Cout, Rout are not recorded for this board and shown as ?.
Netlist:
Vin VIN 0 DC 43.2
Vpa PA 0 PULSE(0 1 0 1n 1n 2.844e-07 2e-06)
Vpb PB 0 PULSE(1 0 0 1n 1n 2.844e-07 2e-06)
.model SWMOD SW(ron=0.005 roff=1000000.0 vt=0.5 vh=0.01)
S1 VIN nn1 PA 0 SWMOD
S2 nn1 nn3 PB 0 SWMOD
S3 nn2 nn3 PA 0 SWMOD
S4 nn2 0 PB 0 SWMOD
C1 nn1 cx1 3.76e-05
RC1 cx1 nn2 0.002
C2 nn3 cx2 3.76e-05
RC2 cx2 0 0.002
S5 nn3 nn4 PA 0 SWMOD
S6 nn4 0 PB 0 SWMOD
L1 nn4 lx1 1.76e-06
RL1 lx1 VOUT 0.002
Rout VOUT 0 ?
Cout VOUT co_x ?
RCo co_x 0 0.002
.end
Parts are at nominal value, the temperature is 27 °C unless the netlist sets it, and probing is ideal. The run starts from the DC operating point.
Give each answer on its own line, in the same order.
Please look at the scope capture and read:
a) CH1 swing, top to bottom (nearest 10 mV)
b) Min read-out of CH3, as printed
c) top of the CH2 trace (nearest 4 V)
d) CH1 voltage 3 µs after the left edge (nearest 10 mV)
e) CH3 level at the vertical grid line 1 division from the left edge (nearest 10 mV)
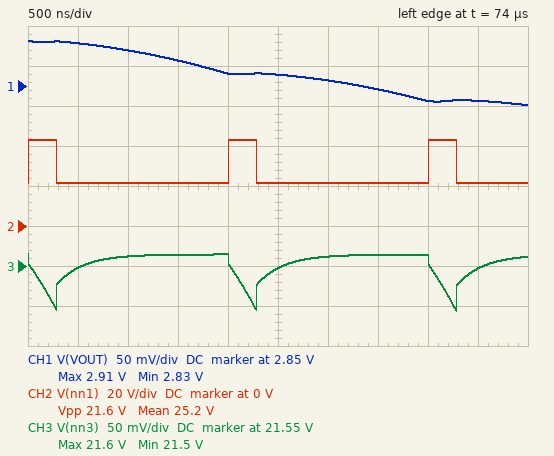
80 mV
21.5 V
44 V
2.86 V
21.55 V
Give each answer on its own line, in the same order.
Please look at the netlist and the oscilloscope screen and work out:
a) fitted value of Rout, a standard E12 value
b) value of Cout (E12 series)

0.18 Ω
100 µF
